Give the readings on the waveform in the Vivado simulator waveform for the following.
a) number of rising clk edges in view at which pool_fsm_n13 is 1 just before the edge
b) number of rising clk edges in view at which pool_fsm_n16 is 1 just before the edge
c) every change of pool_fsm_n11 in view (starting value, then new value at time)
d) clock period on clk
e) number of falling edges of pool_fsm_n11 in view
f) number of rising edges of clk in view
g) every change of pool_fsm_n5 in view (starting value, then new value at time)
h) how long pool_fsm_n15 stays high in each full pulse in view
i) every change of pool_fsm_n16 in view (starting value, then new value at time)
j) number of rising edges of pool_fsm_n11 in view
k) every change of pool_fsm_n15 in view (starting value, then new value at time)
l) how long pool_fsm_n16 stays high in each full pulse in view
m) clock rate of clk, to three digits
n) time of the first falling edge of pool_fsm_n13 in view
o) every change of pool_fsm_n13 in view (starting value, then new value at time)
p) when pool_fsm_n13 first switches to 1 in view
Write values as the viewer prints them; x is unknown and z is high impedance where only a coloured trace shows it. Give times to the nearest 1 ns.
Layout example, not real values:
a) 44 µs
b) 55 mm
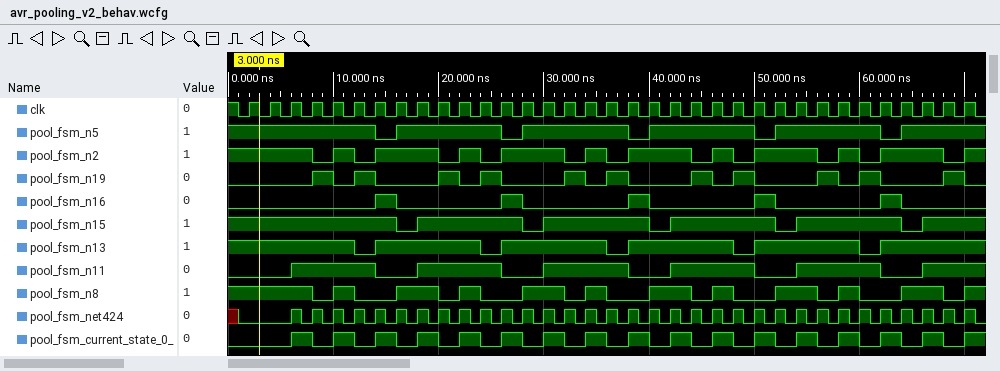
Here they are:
a) 30
b) 5
c) 0, 1 at 6 ns, 0 at 14 ns, 1 at 18 ns, 0 at 26 ns, 1 at 30 ns, 0 at 38 ns, 1 at 42 ns, 0 at 50 ns, 1 at 54 ns, 0 at 62 ns, 1 at 66 ns
d) 2 ns
e) 5
f) 35
g) 1, 0 at 14 ns, 1 at 16 ns, 0 at 26 ns, 1 at 28 ns, 0 at 38 ns, 1 at 40 ns, 0 at 50 ns, 1 at 52 ns, 0 at 62 ns, 1 at 64 ns
h) 10 ns, 10 ns, 10 ns, 10 ns
i) 0, 1 at 14 ns, 0 at 16 ns, 1 at 26 ns, 0 at 28 ns, 1 at 38 ns, 0 at 40 ns, 1 at 50 ns, 0 at 52 ns, 1 at 62 ns, 0 at 64 ns
j) 6
k) 1, 0 at 16 ns, 1 at 18 ns, 0 at 28 ns, 1 at 30 ns, 0 at 40 ns, 1 at 42 ns, 0 at 52 ns, 1 at 54 ns, 0 at 64 ns, 1 at 66 ns
l) 2 ns, 2 ns, 2 ns, 2 ns, 2 ns
m) 500 MHz
n) 12 ns
o) 1, 0 at 12 ns, 1 at 14 ns, 0 at 24 ns, 1 at 26 ns, 0 at 36 ns, 1 at 38 ns, 0 at 48 ns, 1 at 50 ns, 0 at 60 ns, 1 at 62 ns
p) 14 ns
